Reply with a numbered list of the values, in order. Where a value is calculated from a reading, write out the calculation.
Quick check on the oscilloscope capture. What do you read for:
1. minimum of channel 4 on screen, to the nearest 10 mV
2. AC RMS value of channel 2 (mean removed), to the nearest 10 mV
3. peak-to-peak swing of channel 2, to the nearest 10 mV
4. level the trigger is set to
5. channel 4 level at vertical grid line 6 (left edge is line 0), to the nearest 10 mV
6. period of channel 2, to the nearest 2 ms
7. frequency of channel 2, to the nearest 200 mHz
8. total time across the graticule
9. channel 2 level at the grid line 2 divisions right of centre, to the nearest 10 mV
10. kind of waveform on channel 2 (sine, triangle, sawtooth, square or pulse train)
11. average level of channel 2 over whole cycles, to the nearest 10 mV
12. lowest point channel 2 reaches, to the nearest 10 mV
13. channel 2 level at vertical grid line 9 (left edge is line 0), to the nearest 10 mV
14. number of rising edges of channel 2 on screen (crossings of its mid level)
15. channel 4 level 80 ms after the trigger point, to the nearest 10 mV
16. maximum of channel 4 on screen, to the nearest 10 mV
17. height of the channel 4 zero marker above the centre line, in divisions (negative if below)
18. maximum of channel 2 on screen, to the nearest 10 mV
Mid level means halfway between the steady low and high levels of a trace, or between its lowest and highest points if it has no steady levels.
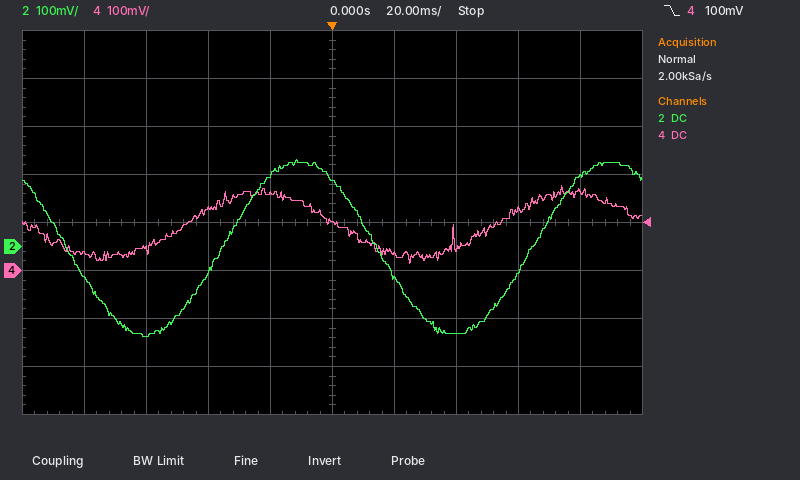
1. 10 mV
2. 370 mV / (2√2) ≈ 131 mV, so 130 mV to the nearest 10 mV
3. 180 mV − (-190 mV) = 370 mV
4. 100 mV
5. 30 mV
6. 100 ms
7. 1 / 100 ms ≈ 10.0 Hz
8. 200 ms
9. -180 mV
10. sine
11. (180 mV + (-190 mV)) / 2 ≈ 0 mV
12. -190 mV
13. 150 mV
14. 2
15. 160 mV
16. 180 mV
17. -1.0 div
18. 180 mV
